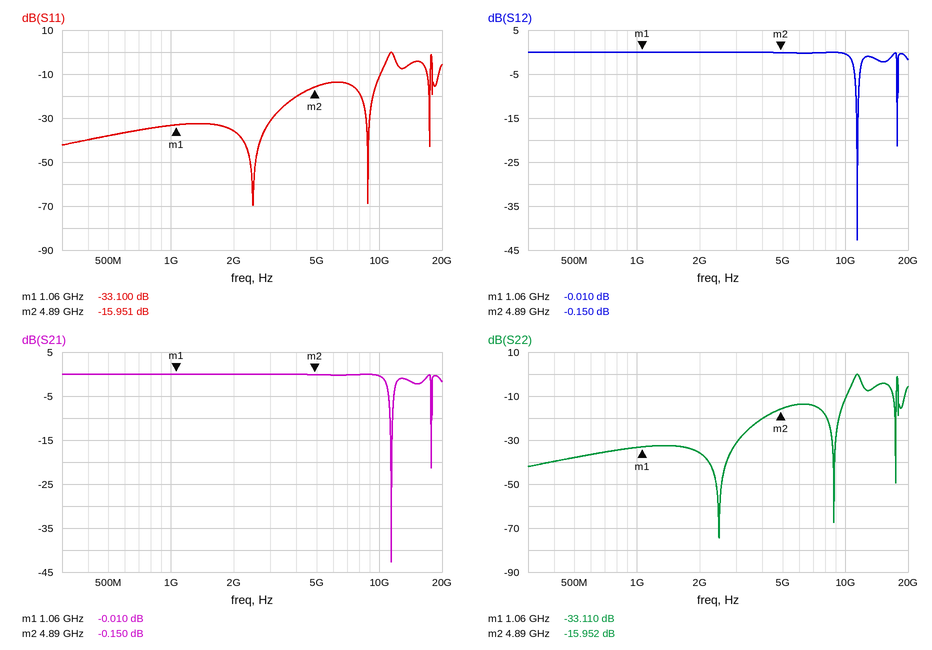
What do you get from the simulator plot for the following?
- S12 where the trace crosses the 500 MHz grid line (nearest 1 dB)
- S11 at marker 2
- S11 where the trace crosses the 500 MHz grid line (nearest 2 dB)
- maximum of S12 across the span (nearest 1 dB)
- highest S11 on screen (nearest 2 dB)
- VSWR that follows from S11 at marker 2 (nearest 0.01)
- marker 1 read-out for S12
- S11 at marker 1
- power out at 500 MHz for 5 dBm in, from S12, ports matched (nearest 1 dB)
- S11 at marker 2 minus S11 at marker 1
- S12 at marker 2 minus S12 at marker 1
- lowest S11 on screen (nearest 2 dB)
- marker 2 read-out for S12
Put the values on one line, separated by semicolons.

0 dB; -15.951 dB; -38 dB; 0 dB; 0 dB; 1.38; -0.010 dB; -33.100 dB; 5 dBm; 17.149 dB; -0.140 dB; -70 dB; -0.150 dB
